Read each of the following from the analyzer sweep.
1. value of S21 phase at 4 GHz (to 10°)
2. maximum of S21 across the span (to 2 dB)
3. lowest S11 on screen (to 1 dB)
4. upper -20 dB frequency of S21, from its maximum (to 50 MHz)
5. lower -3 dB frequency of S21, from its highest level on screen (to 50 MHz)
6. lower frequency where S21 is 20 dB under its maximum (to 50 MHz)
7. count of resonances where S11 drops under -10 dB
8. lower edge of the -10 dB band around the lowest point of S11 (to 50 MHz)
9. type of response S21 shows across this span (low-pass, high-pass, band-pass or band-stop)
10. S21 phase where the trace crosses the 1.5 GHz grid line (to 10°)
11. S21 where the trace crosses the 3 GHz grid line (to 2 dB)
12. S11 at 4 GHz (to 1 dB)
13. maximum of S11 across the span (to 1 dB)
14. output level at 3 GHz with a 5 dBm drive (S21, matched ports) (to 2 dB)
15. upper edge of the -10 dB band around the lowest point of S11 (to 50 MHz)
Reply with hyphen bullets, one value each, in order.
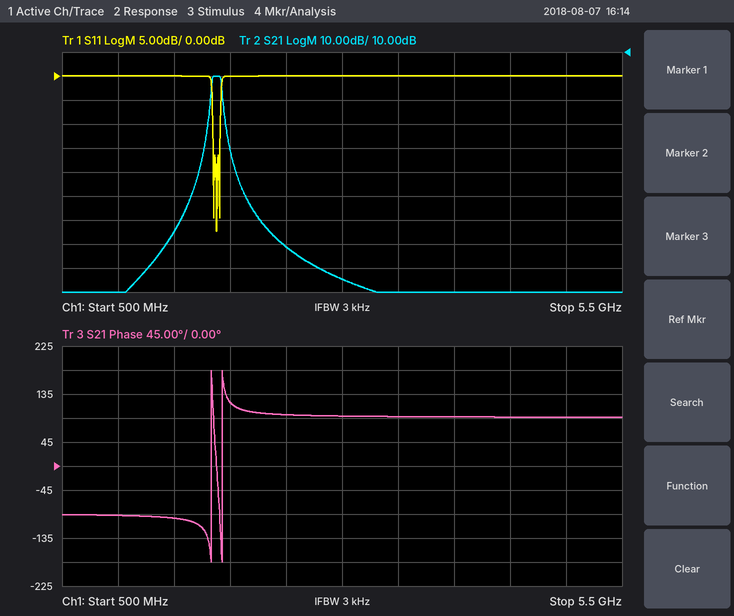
- 90°
- 0 dB
- -32 dB
- 1.95 GHz
- 1.85 GHz
- 1.80 GHz
- 3
- 1.85 GHz
- band-pass
- -100°
- -84 dB
- 0 dB
- 0 dB
- -80 dBm
- 1.90 GHz
